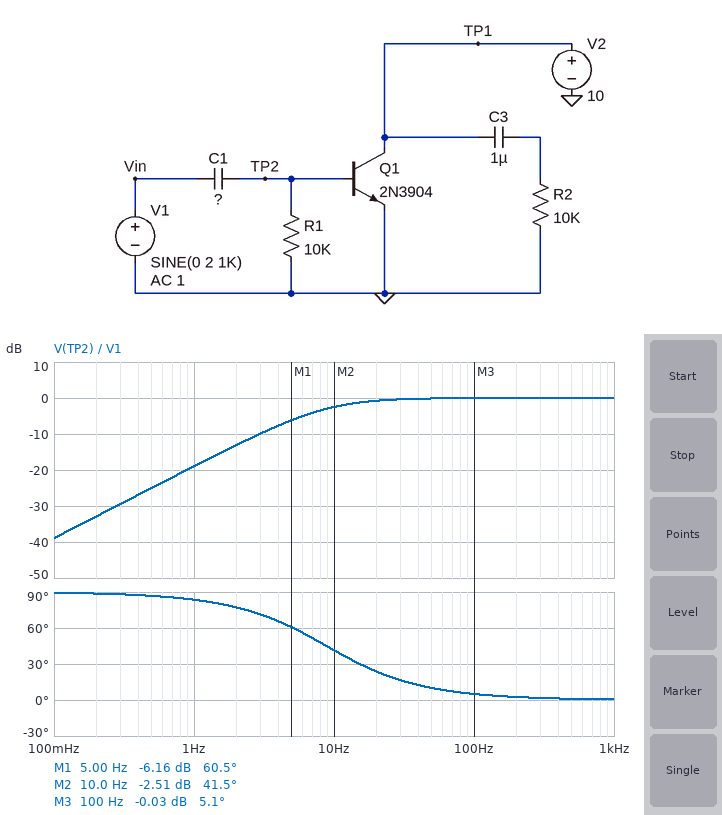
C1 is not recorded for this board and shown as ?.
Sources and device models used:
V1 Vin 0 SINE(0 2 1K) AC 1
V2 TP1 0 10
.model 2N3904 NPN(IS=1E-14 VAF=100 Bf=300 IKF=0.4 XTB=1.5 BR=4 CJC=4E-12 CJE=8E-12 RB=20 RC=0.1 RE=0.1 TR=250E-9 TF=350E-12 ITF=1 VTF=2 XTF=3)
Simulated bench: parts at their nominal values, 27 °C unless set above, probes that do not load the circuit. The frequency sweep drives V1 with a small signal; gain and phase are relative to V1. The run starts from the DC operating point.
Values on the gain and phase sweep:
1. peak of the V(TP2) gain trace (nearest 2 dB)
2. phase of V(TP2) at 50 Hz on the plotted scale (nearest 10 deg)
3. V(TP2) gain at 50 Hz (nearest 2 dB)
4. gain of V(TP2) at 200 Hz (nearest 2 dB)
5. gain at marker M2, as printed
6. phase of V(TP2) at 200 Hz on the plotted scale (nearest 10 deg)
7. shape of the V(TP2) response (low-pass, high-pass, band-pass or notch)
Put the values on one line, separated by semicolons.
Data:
0 dB; 10 deg; 0 dB; 0 dB; -2.51 dB; 0 deg; high-pass
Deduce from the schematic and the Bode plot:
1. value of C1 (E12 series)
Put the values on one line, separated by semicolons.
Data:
1.8 µF
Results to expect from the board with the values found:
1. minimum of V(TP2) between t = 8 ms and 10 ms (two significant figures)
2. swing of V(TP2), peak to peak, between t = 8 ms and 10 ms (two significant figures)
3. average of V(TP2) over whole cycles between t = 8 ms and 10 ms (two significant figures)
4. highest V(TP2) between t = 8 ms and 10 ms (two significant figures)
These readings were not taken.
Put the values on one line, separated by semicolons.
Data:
-3.1 V; 4.0 V; -1.1 V; 880 mV
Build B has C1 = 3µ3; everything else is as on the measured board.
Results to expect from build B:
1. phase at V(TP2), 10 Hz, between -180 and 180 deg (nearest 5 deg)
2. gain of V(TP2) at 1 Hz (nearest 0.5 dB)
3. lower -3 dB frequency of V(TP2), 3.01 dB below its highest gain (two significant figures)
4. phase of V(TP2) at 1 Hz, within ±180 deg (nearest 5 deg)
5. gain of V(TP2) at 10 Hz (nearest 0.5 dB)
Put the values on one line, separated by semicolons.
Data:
25 deg; -14.0 dB; 4.8 Hz; 80 deg; -1.0 dB
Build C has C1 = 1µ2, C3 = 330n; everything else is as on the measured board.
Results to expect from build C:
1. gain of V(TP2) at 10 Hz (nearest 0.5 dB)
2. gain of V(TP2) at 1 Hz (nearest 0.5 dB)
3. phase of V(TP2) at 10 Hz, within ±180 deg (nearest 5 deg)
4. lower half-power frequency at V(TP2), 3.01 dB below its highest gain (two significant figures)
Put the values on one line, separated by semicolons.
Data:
-4.5 dB; -22.5 dB; 55 deg; 13 Hz
